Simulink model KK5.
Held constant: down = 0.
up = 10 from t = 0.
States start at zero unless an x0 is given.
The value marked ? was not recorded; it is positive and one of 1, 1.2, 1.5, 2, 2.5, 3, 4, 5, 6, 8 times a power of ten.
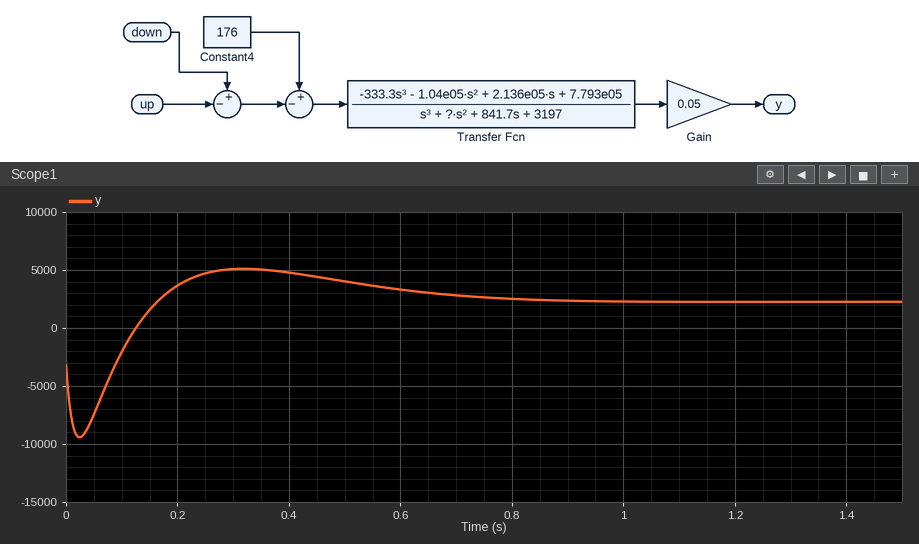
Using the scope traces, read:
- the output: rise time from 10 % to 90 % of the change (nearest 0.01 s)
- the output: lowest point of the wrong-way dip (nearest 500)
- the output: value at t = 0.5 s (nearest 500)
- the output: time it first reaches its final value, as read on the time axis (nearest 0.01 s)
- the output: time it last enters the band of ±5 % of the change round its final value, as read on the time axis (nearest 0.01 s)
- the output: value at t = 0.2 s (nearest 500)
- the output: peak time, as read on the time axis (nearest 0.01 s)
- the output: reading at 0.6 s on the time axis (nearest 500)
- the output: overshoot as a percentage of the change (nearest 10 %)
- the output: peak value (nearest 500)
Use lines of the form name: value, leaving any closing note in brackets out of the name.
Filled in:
the output: rise time from 10 % to 90 % of the change: 0.06 s
the output: lowest point of the wrong-way dip: -9500
the output: value at t = 0.5 s: 4000
the output: time it first reaches its final value, as read on the time axis: 0.16 s
the output: time it last enters the band of ±5 % of the change round its final value, as read on the time axis: 0.79 s
the output: value at t = 0.2 s: 3500
the output: peak time, as read on the time axis: 0.32 s
the output: reading at 0.6 s on the time axis: 3500
the output: overshoot as a percentage of the change: 50 %
the output: peak value: 5000
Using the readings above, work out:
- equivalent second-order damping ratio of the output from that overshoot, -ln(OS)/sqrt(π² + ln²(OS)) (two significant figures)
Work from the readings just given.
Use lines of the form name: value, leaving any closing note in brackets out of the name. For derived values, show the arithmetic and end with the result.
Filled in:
equivalent second-order damping ratio of the output from that overshoot, -ln(OS)/sqrt(π² + ln²(OS)): ln(0.5) = -0.693; 0.693 / sqrt(9.870 + 0.480) = 0.22
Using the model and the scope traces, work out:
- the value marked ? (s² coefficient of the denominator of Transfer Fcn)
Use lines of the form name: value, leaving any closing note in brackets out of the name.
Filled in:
the value marked ?: 80
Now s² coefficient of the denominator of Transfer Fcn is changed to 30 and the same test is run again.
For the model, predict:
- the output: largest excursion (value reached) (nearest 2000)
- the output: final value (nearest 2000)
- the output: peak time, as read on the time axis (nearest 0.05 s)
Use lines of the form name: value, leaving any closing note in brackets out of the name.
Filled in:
the output: largest excursion (value reached): 10000
the output: final value: 2000
the output: peak time, as read on the time axis: 0.15 s
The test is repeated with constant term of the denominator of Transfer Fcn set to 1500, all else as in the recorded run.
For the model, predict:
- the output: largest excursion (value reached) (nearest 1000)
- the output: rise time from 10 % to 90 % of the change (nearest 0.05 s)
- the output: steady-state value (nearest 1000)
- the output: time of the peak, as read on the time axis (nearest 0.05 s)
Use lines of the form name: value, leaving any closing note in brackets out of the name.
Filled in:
the output: largest excursion (value reached): 5000
the output: rise time from 10 % to 90 % of the change: 0.15 s
the output: steady-state value: 5000
the output: time of the peak, as read on the time axis: 0.55 s
